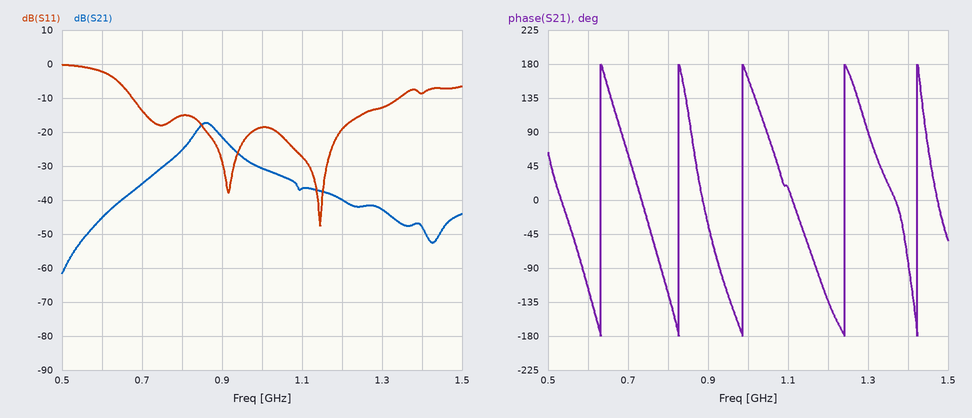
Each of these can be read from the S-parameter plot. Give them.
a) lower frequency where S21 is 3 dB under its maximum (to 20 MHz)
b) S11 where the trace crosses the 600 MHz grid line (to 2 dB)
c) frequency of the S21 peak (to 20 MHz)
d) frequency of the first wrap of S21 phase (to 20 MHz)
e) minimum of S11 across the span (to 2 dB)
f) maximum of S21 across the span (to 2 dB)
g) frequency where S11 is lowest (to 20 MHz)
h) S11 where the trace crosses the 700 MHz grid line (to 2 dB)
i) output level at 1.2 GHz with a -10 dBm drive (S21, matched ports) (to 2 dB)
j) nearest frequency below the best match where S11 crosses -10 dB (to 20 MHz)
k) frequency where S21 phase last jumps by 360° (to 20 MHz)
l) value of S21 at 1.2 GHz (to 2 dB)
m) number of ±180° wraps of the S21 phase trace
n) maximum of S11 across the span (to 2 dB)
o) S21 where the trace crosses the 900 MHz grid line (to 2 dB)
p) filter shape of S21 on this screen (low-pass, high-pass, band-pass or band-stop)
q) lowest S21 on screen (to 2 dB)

840 MHz
-2 dB
860 MHz
640 MHz
-48 dB
-18 dB
1.14 GHz
-14 dB
-50 dBm
680 MHz
1.42 GHz
-40 dB
5
0 dB
-22 dB
band-pass
-62 dB
